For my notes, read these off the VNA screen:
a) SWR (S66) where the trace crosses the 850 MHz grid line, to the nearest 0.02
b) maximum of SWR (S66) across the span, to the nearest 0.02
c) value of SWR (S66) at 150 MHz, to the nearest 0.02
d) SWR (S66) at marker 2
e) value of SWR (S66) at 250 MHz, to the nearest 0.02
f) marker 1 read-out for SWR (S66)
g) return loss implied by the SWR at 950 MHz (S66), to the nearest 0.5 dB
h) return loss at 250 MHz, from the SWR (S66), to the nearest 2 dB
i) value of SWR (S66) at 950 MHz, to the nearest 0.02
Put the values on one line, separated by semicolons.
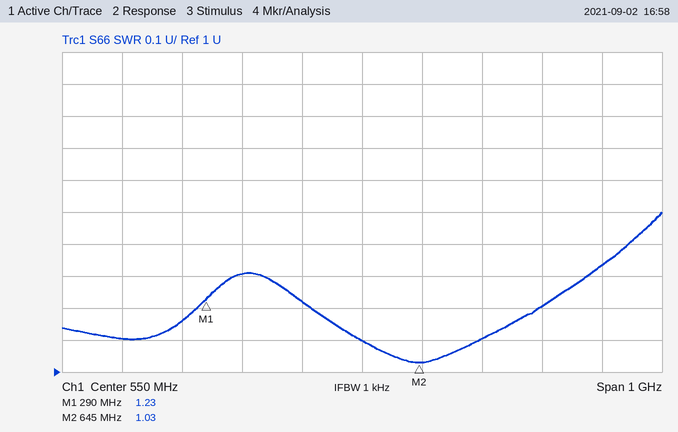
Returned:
1.20; 1.50; 1.10; 1.03; 1.16; 1.23; 17.0 dB; 22 dB; 1.34
